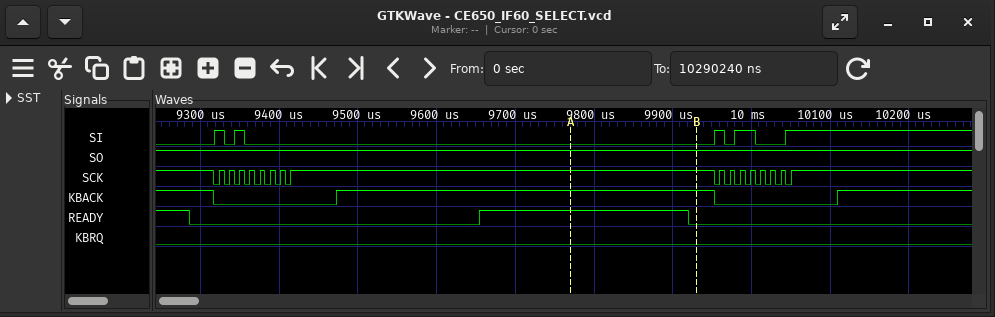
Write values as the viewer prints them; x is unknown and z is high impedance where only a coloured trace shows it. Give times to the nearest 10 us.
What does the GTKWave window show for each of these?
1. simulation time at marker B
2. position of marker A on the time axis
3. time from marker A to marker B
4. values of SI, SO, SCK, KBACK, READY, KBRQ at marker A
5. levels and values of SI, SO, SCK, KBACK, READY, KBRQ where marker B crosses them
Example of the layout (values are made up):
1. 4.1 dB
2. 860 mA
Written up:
1. 9930 us
2. 9770 us
3. 160 us
4. SI=0, SO=1, SCK=1, KBACK=1, READY=1, KBRQ=0
5. SI=0, SO=1, SCK=1, KBACK=1, READY=0, KBRQ=0
